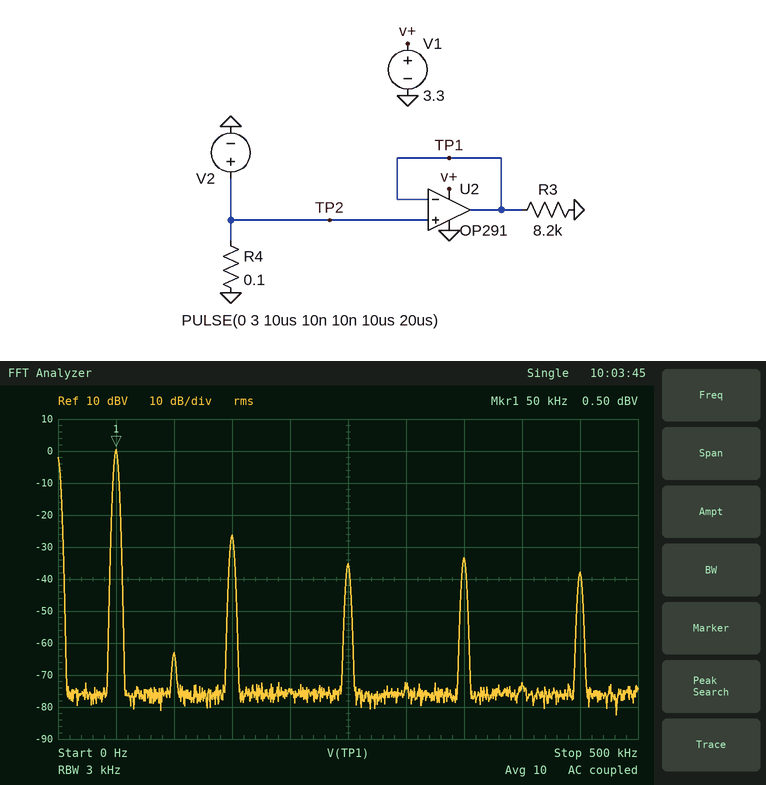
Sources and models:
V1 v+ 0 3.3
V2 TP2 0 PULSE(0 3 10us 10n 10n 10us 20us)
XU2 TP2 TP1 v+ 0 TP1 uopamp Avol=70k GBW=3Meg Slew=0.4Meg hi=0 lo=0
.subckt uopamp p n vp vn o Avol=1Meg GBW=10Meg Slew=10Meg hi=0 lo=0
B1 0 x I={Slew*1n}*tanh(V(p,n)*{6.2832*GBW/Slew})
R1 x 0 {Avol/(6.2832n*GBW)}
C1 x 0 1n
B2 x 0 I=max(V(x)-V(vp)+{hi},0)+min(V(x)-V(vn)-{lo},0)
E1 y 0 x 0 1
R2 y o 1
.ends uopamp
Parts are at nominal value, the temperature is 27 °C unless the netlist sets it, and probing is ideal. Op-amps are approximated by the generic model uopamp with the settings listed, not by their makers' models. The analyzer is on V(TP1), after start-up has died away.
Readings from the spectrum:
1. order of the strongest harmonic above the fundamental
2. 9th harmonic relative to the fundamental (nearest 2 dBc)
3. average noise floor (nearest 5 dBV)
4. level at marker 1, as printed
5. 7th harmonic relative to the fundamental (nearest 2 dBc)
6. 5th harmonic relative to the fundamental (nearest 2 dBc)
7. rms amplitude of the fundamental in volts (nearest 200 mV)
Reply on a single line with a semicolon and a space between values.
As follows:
3; -38 dBc; -75 dBV; 0.50 dBV; -34 dBc; -36 dBc; 1.0 V
